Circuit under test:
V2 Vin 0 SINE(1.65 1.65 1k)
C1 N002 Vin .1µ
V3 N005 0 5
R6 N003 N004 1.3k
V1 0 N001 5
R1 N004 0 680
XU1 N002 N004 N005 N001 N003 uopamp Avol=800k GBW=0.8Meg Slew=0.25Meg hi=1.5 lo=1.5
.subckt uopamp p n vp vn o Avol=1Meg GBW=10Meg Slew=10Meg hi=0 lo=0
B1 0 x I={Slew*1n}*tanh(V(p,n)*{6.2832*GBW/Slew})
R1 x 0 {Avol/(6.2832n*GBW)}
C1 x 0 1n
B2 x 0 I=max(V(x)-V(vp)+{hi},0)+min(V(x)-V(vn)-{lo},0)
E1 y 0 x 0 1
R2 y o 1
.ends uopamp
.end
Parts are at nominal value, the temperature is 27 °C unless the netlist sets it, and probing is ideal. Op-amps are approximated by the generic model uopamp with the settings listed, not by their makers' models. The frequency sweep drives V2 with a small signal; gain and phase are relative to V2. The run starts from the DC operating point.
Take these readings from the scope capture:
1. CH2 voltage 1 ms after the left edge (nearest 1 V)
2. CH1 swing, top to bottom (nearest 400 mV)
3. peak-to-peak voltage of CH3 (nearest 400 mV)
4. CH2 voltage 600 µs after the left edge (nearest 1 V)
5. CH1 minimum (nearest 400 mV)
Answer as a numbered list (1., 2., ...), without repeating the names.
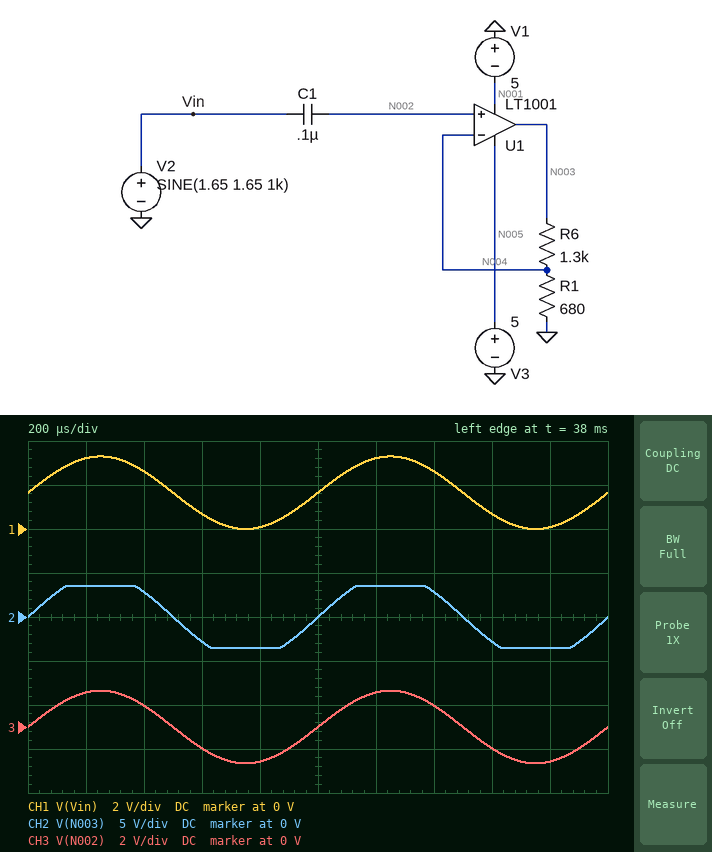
1. 0 V
2. 3.2 V
3. 3.2 V
4. -3 V
5. 0 V
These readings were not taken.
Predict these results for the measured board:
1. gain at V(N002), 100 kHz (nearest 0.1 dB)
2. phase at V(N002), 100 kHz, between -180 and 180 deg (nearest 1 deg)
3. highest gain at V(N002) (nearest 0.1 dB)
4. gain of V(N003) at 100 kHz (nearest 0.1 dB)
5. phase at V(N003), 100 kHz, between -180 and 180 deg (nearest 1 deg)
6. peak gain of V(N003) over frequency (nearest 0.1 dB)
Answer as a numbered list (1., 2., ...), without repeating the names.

1. 0 dB
2. 0 deg
3. 0 dB
4. 8.7 dB
5. -20 deg
6. 9.3 dB
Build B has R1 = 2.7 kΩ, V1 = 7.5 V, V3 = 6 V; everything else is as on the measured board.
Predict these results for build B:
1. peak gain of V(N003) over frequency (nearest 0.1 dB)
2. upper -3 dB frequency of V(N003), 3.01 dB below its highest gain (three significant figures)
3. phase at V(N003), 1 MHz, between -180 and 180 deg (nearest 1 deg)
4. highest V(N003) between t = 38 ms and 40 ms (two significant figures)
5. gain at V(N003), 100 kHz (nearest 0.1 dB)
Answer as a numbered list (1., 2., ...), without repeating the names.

1. 3.4 dB
2. 540 kHz
3. -62 deg
4. 4.5 V
5. 3.3 dB
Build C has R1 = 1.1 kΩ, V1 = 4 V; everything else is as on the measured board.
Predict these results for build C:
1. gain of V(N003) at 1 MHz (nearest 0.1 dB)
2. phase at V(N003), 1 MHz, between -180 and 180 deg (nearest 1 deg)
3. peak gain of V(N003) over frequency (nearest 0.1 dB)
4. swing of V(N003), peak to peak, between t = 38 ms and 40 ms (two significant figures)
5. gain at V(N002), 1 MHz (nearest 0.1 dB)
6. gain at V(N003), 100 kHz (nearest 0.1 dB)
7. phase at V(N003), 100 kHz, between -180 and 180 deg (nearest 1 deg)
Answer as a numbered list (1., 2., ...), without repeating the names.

1. -2.5 dB
2. -70 deg
3. 6.8 dB
4. 3.5 V
5. 0 dB
6. 6.5 dB
7. -15 deg
